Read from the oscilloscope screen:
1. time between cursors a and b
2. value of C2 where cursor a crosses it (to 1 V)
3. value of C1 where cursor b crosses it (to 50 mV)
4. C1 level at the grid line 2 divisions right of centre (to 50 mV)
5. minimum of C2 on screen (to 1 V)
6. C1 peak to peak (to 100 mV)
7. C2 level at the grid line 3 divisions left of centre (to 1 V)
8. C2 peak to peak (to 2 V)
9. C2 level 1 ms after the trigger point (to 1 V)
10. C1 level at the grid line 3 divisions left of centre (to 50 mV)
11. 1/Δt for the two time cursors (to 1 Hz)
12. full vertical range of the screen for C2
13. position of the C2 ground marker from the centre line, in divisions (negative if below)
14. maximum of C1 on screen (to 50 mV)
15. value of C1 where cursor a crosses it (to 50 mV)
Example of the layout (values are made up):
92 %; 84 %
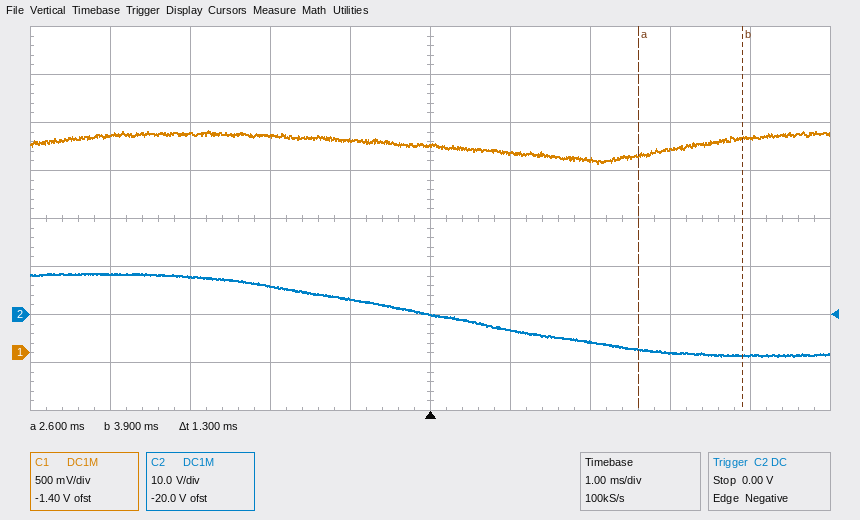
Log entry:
1.3 ms; -7 V; 2.25 V; 2.00 V; -9 V; 300 mV; 8 V; 18 V; -3 V; 2.30 V; 769 Hz; 80 V; -2.0 div; 2.30 V; 2.05 V
